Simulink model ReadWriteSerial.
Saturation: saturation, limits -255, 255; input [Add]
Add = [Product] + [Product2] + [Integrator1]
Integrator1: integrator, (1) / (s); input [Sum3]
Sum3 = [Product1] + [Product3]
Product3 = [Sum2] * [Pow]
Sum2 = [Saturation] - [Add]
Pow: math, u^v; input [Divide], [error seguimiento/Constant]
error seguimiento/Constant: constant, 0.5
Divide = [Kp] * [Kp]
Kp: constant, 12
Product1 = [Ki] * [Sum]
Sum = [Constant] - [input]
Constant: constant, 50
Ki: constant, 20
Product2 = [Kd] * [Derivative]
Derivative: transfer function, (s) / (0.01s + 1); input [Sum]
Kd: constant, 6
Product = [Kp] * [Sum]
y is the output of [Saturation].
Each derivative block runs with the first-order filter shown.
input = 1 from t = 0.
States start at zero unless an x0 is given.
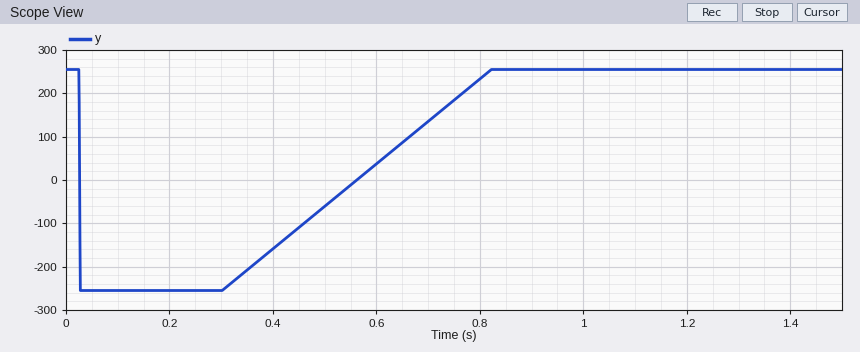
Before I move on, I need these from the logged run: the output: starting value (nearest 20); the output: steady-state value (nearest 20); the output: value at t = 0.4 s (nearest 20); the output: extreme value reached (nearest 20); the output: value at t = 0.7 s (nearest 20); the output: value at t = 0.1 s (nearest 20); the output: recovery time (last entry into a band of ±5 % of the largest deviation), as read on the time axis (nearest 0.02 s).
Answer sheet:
260
260
-160
-260
140
-260
0.80 s
